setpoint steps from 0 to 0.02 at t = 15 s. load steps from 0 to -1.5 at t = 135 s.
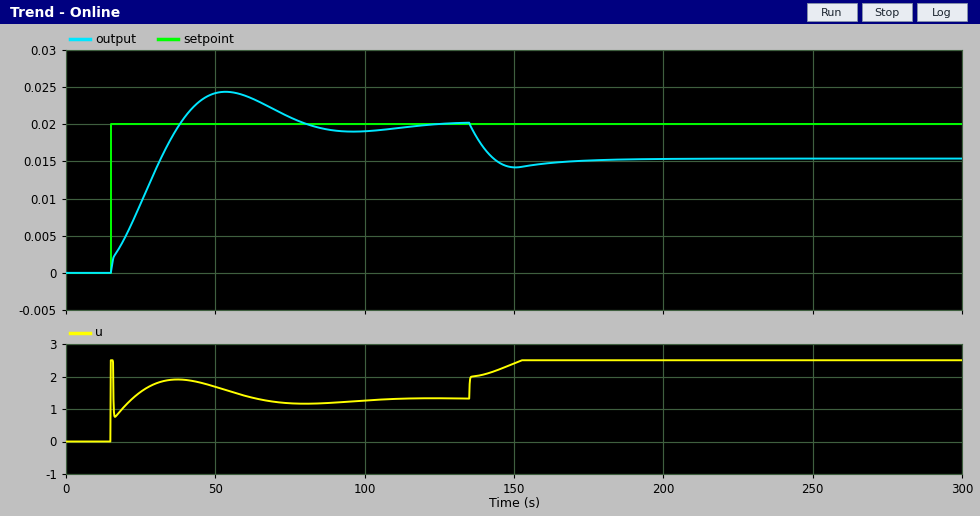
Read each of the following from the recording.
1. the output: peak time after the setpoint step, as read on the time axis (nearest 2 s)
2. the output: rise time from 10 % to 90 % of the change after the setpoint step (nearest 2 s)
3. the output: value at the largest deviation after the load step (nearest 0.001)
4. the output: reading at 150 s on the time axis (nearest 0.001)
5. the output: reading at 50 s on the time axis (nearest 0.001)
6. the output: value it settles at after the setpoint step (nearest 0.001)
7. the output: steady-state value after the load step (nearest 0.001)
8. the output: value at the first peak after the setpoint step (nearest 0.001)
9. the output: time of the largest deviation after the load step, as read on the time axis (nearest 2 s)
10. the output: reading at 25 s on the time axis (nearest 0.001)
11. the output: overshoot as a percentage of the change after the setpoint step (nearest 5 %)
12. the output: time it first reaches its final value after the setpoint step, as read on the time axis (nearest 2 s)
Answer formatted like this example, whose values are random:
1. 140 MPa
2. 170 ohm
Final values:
1. 54 s
2. 20 s
3. 0.014
4. 0.014
5. 0.024
6. 0.020
7. 0.015
8. 0.024
9. 150 s
10. 0.009
11. 20 %
12. 38 s
